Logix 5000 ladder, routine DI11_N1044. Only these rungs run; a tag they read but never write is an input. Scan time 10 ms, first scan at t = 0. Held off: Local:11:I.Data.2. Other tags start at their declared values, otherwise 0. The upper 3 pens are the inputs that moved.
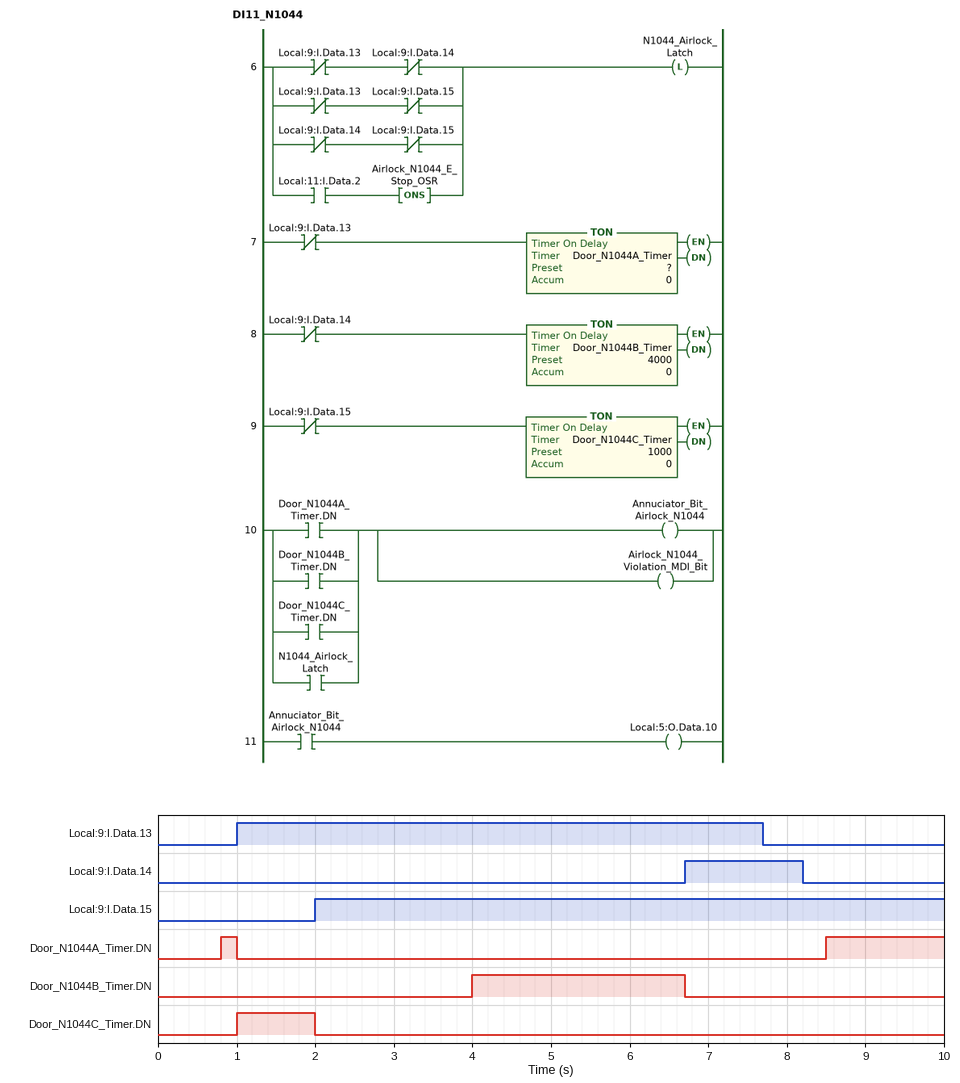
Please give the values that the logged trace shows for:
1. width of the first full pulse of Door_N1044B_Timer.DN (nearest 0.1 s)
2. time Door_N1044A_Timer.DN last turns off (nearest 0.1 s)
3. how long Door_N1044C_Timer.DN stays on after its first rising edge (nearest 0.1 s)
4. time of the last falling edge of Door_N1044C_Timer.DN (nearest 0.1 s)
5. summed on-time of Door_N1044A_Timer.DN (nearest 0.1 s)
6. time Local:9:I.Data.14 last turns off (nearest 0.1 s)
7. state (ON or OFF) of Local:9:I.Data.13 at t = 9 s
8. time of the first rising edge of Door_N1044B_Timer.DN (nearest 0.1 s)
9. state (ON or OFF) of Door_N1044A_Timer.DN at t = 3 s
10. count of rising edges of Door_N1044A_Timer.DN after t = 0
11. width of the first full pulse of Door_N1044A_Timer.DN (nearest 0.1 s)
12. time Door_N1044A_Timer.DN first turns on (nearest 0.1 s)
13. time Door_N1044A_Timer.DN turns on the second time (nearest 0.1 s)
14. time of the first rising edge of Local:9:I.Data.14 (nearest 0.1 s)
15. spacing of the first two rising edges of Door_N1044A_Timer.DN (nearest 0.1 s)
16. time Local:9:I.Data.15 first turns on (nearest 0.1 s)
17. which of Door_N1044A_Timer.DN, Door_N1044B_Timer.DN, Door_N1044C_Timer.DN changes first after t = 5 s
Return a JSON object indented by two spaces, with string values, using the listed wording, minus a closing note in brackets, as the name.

{
  "width of the first full pulse of Door_N1044B_Timer.DN": "2.7 s",
  "time Door_N1044A_Timer.DN last turns off": "1.0 s",
  "how long Door_N1044C_Timer.DN stays on after its first rising edge": "1.0 s",
  "time of the last falling edge of Door_N1044C_Timer.DN": "2.0 s",
  "summed on-time of Door_N1044A_Timer.DN": "1.7 s",
  "time Local:9:I.Data.14 last turns off": "8.2 s",
  "state (ON or OFF) of Local:9:I.Data.13 at t = 9 s": "OFF",
  "time of the first rising edge of Door_N1044B_Timer.DN": "4.0 s",
  "state (ON or OFF) of Door_N1044A_Timer.DN at t = 3 s": "OFF",
  "count of rising edges of Door_N1044A_Timer.DN after t = 0": "2",
  "width of the first full pulse of Door_N1044A_Timer.DN": "0.2 s",
  "time Door_N1044A_Timer.DN first turns on": "0.8 s",
  "time Door_N1044A_Timer.DN turns on the second time": "8.5 s",
  "time of the first rising edge of Local:9:I.Data.14": "6.7 s",
  "spacing of the first two rising edges of Door_N1044A_Timer.DN": "7.7 s",
  "time Local:9:I.Data.15 first turns on": "2.0 s",
  "which of Door_N1044A_Timer.DN, Door_N1044B_Timer.DN, Door_N1044C_Timer.DN changes first after t = 5 s": "Door_N1044B_Timer.DN"
}
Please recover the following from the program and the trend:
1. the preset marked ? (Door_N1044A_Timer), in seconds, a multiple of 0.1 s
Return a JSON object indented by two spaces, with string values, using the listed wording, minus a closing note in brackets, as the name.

{
  "the preset marked ? (Door_N1044A_Timer), in seconds, a multiple of 0.1 s": "0.8 s"
}
